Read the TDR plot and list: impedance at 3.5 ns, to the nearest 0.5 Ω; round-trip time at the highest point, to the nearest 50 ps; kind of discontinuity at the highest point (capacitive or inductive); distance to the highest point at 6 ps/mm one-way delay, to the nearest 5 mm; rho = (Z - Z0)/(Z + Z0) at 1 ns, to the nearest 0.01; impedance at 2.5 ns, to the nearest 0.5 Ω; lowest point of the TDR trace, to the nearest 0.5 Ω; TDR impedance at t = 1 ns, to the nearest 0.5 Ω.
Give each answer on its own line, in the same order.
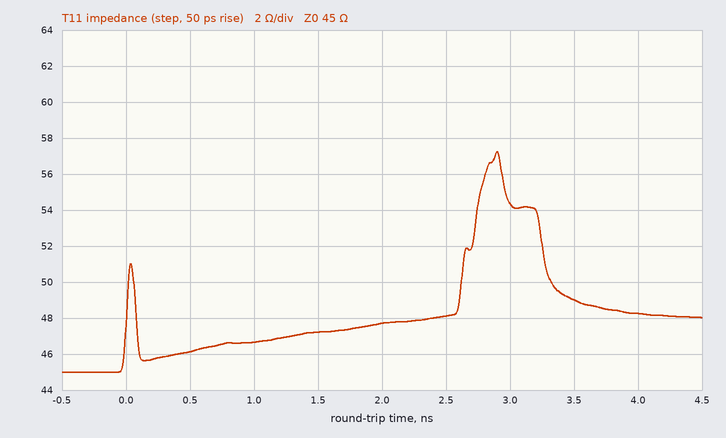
49.0 Ω
2.90 ns
inductive
240 mm
+0.02
48.0 Ω
45.0 Ω
46.5 Ω
